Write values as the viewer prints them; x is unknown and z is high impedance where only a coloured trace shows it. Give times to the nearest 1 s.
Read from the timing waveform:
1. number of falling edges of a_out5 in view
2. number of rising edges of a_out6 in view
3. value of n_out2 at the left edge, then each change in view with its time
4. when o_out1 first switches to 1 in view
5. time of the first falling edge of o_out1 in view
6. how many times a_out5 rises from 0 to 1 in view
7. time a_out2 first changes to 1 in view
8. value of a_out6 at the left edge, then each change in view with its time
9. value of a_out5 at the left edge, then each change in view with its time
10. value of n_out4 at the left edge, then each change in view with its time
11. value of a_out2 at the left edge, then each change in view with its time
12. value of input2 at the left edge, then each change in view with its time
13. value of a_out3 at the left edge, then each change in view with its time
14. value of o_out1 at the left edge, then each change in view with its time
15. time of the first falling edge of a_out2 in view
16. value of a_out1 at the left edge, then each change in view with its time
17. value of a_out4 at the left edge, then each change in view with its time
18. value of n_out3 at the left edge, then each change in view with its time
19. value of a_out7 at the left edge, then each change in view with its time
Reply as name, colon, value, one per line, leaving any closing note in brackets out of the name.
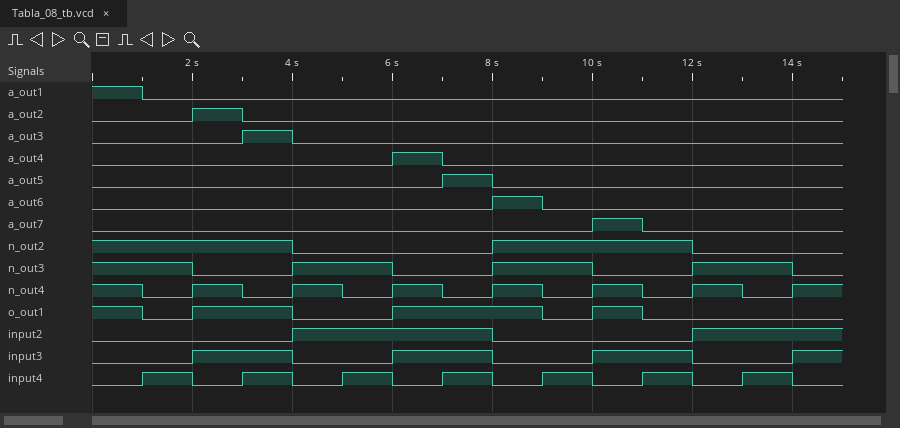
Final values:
number of falling edges of a_out5 in view: 1
number of rising edges of a_out6 in view: 1
value of n_out2 at the left edge, then each change in view with its time: 1, 0 at 4 s, 1 at 8 s, 0 at 12 s
when o_out1 first switches to 1 in view: 2 s
time of the first falling edge of o_out1 in view: 1 s
how many times a_out5 rises from 0 to 1 in view: 1
time a_out2 first changes to 1 in view: 2 s
value of a_out6 at the left edge, then each change in view with its time: 0, 1 at 8 s, 0 at 9 s
value of a_out5 at the left edge, then each change in view with its time: 0, 1 at 7 s, 0 at 8 s
value of n_out4 at the left edge, then each change in view with its time: 1, 0 at 1 s, 1 at 2 s, 0 at 3 s, 1 at 4 s, 0 at 5 s, 1 at 6 s, 0 at 7 s, 1 at 8 s, 0 at 9 s, 1 at 10 s, 0 at 11 s, 1 at 12 s, 0 at 13 s, 1 at 14 s
value of a_out2 at the left edge, then each change in view with its time: 0, 1 at 2 s, 0 at 3 s
value of input2 at the left edge, then each change in view with its time: 0, 1 at 4 s, 0 at 8 s, 1 at 12 s
value of a_out3 at the left edge, then each change in view with its time: 0, 1 at 3 s, 0 at 4 s
value of o_out1 at the left edge, then each change in view with its time: 1, 0 at 1 s, 1 at 2 s, 0 at 4 s, 1 at 6 s, 0 at 9 s, 1 at 10 s, 0 at 11 s
time of the first falling edge of a_out2 in view: 3 s
value of a_out1 at the left edge, then each change in view with its time: 1, 0 at 1 s
value of a_out4 at the left edge, then each change in view with its time: 0, 1 at 6 s, 0 at 7 s
value of n_out3 at the left edge, then each change in view with its time: 1, 0 at 2 s, 1 at 4 s, 0 at 6 s, 1 at 8 s, 0 at 10 s, 1 at 12 s, 0 at 14 s
value of a_out7 at the left edge, then each change in view with its time: 0, 1 at 10 s, 0 at 11 s
